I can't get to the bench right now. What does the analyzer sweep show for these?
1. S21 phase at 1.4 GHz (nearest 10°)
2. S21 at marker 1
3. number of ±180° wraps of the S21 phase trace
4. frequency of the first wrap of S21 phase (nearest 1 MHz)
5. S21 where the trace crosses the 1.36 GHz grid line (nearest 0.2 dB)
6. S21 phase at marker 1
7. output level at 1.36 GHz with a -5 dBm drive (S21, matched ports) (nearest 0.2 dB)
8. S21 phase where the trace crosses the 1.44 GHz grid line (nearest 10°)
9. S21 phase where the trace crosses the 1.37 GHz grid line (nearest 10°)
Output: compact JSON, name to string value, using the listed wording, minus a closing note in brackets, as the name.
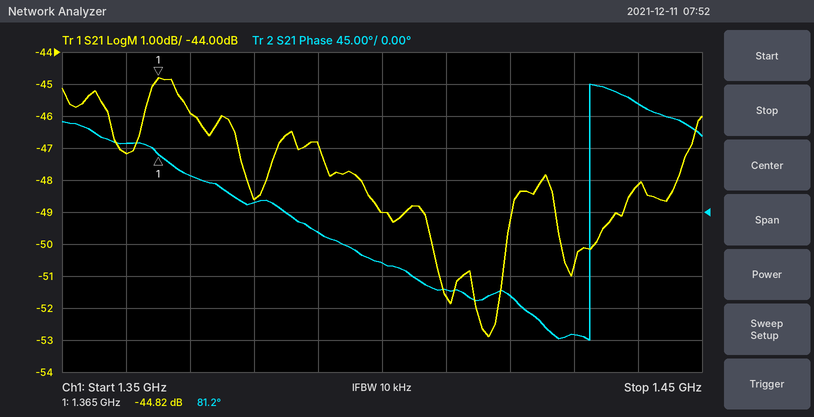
{"S21 phase at 1.4 GHz": "-70°", "S21 at marker 1": "-44.82 dB", "number of ±180° wraps of the S21 phase trace": "1", "frequency of the first wrap of S21 phase": "1.432 GHz", "S21 where the trace crosses the 1.36 GHz grid line": "-47.2 dB", "S21 phase at marker 1": "81.2°", "output level at 1.36 GHz with a -5 dBm drive (S21, matched ports)": "-52.2 dBm", "S21 phase where the trace crosses the 1.44 GHz grid line": "150°", "S21 phase where the trace crosses the 1.37 GHz grid line": "50°"}
